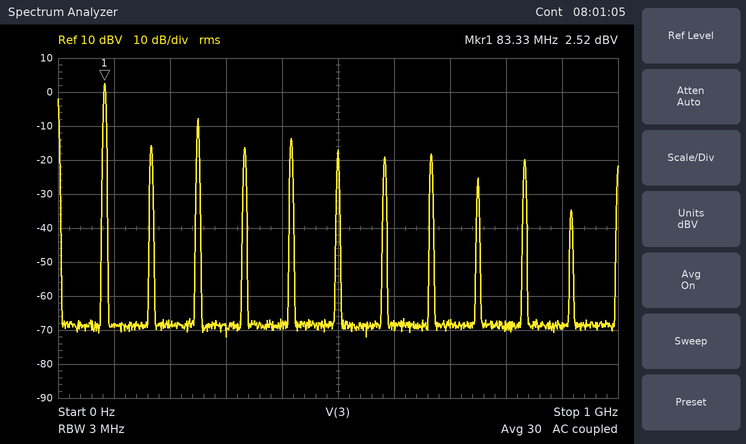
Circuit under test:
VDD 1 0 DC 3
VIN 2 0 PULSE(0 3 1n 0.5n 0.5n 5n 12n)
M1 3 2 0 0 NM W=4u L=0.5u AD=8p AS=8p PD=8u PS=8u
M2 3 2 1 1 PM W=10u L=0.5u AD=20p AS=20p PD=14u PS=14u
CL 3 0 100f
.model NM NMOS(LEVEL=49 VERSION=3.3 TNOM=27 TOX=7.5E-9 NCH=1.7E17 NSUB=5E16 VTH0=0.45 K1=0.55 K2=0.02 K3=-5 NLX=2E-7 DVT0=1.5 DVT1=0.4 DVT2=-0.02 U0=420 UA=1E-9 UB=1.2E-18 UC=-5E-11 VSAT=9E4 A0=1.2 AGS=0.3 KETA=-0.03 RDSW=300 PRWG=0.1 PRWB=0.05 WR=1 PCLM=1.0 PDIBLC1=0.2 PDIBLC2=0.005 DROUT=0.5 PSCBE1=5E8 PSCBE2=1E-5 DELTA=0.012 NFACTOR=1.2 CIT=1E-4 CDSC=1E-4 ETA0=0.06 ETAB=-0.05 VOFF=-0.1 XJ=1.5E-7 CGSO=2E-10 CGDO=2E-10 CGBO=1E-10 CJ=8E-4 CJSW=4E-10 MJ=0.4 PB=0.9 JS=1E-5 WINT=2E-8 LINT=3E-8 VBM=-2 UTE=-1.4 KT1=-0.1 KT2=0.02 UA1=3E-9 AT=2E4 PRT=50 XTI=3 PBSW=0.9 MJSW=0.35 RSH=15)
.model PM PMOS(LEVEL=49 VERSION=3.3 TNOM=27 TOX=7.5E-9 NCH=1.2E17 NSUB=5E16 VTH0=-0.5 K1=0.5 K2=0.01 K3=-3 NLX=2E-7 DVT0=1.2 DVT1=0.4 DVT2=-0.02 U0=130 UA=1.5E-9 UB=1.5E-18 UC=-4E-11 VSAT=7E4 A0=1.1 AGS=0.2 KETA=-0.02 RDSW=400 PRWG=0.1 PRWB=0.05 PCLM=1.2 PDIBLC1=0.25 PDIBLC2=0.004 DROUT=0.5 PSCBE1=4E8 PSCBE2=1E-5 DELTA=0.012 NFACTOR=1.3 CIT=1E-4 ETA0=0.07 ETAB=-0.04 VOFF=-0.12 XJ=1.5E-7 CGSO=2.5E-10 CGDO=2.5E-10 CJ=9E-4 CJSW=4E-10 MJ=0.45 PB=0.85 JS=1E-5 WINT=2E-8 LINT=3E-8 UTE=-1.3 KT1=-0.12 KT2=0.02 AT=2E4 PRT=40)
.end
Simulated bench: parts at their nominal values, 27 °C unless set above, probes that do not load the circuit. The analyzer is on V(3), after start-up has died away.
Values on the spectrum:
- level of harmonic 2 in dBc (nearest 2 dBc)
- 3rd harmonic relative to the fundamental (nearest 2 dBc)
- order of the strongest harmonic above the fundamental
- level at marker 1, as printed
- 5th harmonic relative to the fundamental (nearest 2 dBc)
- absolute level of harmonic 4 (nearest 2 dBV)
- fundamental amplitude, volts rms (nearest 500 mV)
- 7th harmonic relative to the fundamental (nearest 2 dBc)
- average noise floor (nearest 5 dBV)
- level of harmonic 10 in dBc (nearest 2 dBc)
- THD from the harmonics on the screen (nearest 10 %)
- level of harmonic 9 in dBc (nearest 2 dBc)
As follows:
-18 dBc
-10 dBc
3
2.52 dBV
-16 dBc
-16 dBV
1.5 V
-22 dBc
-70 dBV
-22 dBc
40 %
-28 dBc
